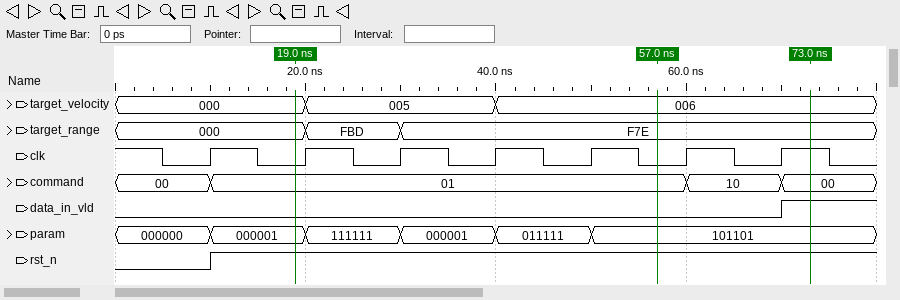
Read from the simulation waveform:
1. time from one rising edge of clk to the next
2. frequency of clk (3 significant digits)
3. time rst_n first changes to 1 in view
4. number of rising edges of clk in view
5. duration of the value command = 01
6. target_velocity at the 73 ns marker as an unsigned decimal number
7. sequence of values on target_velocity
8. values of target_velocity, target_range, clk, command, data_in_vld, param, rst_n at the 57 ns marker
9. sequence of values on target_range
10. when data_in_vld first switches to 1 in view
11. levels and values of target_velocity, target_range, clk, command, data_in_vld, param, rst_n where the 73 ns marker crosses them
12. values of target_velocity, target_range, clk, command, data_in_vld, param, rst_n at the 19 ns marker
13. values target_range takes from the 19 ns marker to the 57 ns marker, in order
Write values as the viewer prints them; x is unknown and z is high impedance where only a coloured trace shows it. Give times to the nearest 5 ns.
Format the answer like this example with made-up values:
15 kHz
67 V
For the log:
10 ns
100 MHz
10 ns
7
50 ns
6
000, 005, 006
target_velocity=006, target_range=F7E, clk=0, command=01, data_in_vld=0, param=101101, rst_n=1
000, FBD, F7E
70 ns
target_velocity=006, target_range=F7E, clk=1, command=00, data_in_vld=1, param=101101, rst_n=1
target_velocity=000, target_range=000, clk=0, command=01, data_in_vld=0, param=000001, rst_n=1
000, FBD, F7E
